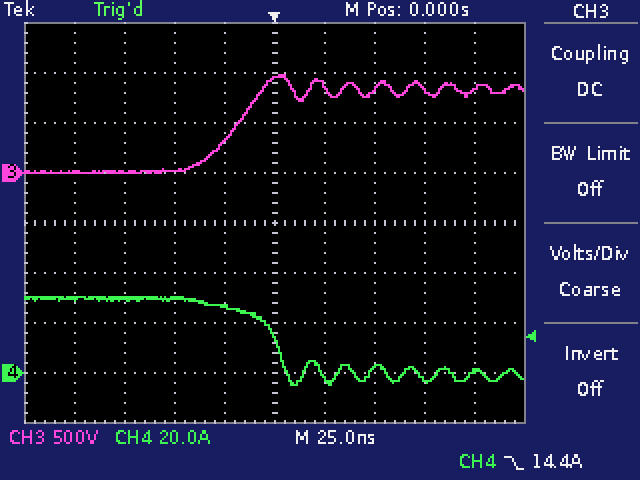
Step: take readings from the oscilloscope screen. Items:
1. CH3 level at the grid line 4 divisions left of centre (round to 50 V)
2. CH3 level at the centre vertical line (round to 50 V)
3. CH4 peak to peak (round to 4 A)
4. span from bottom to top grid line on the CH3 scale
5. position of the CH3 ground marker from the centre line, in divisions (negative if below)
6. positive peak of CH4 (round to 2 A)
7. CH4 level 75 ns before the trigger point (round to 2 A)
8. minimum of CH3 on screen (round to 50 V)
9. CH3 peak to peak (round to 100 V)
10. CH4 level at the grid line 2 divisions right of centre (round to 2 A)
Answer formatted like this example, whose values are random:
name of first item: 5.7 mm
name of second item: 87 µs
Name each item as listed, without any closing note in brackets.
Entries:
CH3 level at the grid line 4 divisions left of centre: 0 V
CH3 level at the centre vertical line: 950 V
CH4 peak to peak: 36 A
span from bottom to top grid line on the CH3 scale: 4 kV
position of the CH3 ground marker from the centre line, in divisions: +1.0 div
positive peak of CH4: 30 A
CH4 level 75 ns before the trigger point: 30 A
minimum of CH3 on screen: 0 V
CH3 peak to peak: 1.00 kV
CH4 level at the grid line 2 divisions right of centre: 2 A
